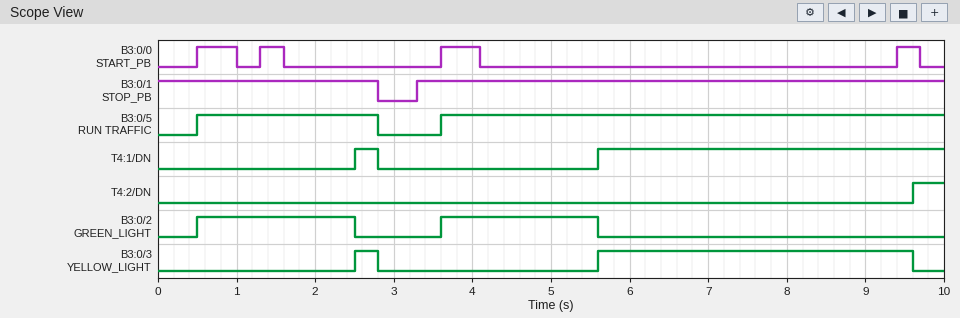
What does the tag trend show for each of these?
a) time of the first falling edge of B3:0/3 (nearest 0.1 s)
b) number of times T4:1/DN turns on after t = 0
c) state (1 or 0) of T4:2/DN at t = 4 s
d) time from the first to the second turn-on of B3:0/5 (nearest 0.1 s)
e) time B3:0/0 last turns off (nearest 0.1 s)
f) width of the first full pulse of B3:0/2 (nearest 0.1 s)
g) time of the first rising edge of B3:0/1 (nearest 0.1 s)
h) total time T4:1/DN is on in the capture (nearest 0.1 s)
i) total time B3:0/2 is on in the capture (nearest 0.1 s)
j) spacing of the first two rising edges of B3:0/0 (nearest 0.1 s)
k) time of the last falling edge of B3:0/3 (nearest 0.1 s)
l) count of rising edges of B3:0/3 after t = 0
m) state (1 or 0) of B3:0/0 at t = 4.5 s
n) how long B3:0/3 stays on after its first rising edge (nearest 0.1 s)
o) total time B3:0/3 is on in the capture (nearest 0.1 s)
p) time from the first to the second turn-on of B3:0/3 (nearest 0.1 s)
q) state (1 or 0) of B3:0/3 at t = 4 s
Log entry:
2.8 s
2
0
3.1 s
9.7 s
2.0 s
3.3 s
4.7 s
4.0 s
0.8 s
9.6 s
2
0
0.3 s
4.3 s
3.1 s
0
